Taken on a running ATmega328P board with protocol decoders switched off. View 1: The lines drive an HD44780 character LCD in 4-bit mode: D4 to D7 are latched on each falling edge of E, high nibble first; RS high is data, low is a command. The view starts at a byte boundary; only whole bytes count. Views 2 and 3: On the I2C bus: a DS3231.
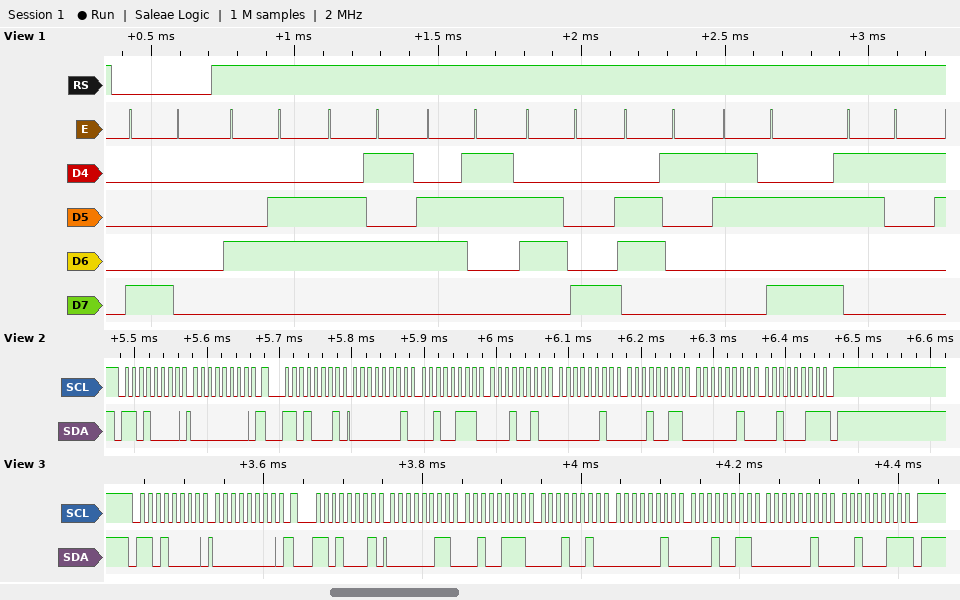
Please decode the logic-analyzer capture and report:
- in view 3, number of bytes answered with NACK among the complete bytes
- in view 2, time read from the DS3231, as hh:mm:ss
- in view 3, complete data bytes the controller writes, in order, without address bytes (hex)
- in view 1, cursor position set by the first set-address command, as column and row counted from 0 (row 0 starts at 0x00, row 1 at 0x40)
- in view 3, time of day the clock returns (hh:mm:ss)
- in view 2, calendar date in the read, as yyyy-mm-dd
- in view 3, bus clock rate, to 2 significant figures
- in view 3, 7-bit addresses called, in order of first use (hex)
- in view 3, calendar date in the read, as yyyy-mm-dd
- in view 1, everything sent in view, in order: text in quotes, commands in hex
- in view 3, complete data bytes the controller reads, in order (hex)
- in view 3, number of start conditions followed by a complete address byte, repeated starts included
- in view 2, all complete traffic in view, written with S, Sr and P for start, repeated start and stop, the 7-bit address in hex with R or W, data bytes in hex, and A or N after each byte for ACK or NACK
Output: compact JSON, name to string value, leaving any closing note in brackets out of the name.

{"in view 3, number of bytes answered with NACK among the complete bytes": "1", "in view 2, time read from the DS3231, as hh:mm:ss": "12:27:01", "in view 3, complete data bytes the controller writes, in order, without address bytes": "00", "in view 1, cursor position set by the first set-address command, as column and row counted from 0": "column 0, row 0", "in view 3, time of day the clock returns": "12:27:03", "in view 2, calendar date in the read, as yyyy-mm-dd": "2023-02-13", "in view 3, bus clock rate, to 2 significant figures": "100 kHz", "in view 3, 7-bit addresses called, in order of first use": "0x68", "in view 3, calendar date in the read, as yyyy-mm-dd": "2023-02-13", "in view 1, everything sent in view, in order: text in quotes, commands in hex": "0x80 \"Fecha:1\"", "in view 3, complete data bytes the controller reads, in order": "03 27 12 02 13 02 23", "in view 3, number of start conditions followed by a complete address byte, repeated starts included": "2", "in view 2, all complete traffic in view, written with S, Sr and P for start, repeated start and stop, the 7-bit address in hex with R or W, data bytes in hex, and A or N after each byte for ACK or NACK": "S 68W A 00 A Sr 68R A 01 A 27 A 12 A 02 A 13 A 02 A 23 N P"}
